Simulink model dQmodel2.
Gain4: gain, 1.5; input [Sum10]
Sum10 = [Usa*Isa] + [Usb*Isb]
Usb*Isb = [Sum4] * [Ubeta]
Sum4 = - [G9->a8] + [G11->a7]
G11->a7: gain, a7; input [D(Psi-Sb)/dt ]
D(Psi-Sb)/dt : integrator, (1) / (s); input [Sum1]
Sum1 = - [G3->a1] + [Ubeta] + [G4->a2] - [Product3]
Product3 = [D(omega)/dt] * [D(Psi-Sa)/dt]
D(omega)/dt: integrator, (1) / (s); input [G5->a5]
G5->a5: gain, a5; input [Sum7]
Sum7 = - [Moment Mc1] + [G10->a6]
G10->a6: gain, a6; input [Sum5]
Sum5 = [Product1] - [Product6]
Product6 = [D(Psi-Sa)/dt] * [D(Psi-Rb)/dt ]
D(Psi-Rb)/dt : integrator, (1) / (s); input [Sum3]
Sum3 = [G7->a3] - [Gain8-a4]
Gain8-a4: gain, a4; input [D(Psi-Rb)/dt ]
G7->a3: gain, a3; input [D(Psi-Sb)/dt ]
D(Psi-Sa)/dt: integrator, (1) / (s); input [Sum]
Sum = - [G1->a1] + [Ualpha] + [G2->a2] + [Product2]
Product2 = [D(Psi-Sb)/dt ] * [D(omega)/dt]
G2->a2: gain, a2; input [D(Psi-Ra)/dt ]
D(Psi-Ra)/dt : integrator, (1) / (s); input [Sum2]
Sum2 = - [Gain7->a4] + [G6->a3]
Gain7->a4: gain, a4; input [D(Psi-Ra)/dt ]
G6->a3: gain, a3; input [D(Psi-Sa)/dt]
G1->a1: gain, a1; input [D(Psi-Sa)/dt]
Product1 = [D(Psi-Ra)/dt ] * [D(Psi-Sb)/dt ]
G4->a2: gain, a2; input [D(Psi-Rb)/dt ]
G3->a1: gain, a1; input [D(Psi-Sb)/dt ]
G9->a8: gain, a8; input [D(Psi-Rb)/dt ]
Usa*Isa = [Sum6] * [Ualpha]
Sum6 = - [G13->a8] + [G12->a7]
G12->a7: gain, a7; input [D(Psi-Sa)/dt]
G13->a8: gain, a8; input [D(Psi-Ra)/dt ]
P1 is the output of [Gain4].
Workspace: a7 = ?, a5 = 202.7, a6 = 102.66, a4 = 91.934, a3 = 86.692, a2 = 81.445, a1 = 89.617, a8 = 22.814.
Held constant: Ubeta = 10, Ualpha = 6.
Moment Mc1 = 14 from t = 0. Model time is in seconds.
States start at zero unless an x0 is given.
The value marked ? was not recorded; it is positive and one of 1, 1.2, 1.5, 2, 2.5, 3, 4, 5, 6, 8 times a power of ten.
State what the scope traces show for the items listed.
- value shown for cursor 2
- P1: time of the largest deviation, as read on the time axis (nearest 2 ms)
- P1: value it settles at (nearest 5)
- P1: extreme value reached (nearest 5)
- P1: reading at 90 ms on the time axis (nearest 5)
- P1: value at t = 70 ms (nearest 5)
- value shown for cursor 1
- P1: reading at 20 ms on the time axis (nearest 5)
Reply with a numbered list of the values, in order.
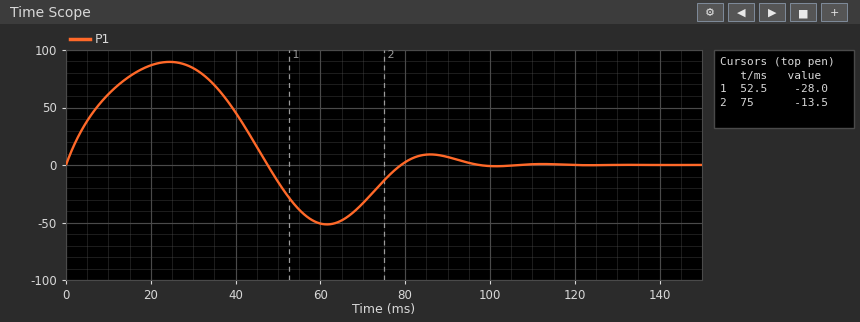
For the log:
1. -13.5
2. 24 ms
3. 0
4. 90
5. 5
6. -35
7. -28.0
8. 85
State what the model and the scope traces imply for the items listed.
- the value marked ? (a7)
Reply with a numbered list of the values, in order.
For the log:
1. 50
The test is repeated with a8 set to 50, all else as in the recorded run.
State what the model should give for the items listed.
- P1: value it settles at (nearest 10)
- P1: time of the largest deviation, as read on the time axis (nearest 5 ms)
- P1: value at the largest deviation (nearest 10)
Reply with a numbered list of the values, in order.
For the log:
1. 0
2. 55 ms
3. -60
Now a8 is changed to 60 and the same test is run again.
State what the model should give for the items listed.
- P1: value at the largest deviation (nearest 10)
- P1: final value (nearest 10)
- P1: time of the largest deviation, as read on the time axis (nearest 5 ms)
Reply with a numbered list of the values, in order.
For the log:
1. -70
2. 0
3. 55 ms
